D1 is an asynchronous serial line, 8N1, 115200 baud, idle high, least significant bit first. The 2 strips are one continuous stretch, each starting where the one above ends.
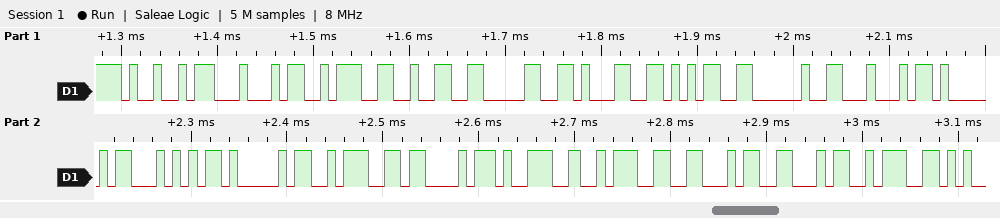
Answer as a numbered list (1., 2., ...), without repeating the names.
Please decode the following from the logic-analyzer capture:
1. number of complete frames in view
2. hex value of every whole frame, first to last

1. 19
2. 49 44 3A 32 30 31 35 20 44 41 54 41 3A 43 39 3A 46 46 3A
